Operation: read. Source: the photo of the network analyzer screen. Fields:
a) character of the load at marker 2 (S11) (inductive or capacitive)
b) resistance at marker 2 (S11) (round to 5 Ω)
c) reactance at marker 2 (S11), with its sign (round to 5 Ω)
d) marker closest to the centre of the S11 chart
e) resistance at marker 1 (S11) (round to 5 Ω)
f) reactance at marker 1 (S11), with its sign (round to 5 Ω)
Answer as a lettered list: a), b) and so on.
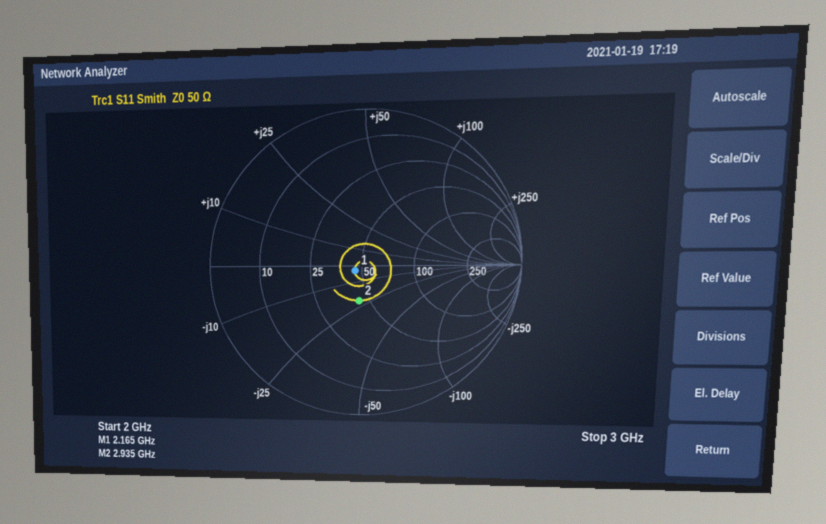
a) capacitive
b) 45 Ω
c) -20 Ω
d) marker 1
e) 45 Ω
f) -5 Ω
